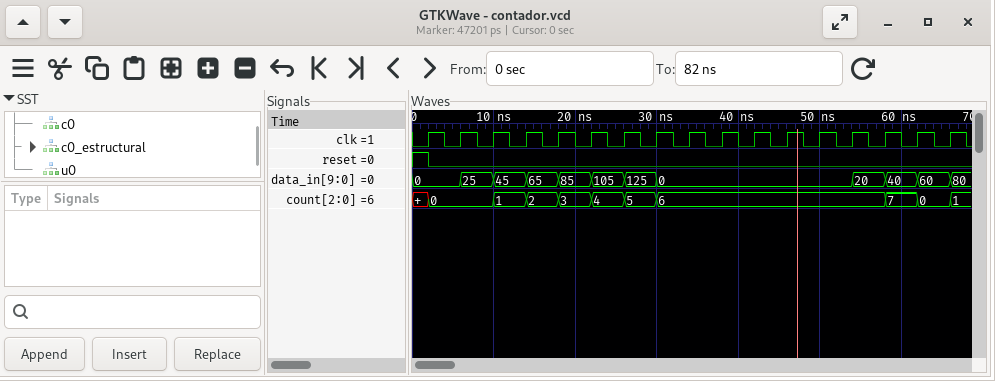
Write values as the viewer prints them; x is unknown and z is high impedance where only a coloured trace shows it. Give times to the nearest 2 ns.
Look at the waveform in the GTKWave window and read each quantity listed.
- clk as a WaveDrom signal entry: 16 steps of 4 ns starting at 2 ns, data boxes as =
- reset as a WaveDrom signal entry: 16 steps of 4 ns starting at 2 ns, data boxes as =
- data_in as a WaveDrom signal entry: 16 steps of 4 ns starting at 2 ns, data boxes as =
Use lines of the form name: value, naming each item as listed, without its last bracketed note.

clk as a WaveDrom signal entry: 16 steps of 4 ns starting at 2 ns, data boxes as =: {name: 'clk', wave: 'p...............'}
reset as a WaveDrom signal entry: 16 steps of 4 ns starting at 2 ns, data boxes as =: {name: 'reset', wave: '0...............'}
data_in as a WaveDrom signal entry: 16 steps of 4 ns starting at 2 ns, data boxes as =: {name: 'data_in', wave: '========.....===', data: '0 25 45 65 85 105 125 0 20 40 60'}
